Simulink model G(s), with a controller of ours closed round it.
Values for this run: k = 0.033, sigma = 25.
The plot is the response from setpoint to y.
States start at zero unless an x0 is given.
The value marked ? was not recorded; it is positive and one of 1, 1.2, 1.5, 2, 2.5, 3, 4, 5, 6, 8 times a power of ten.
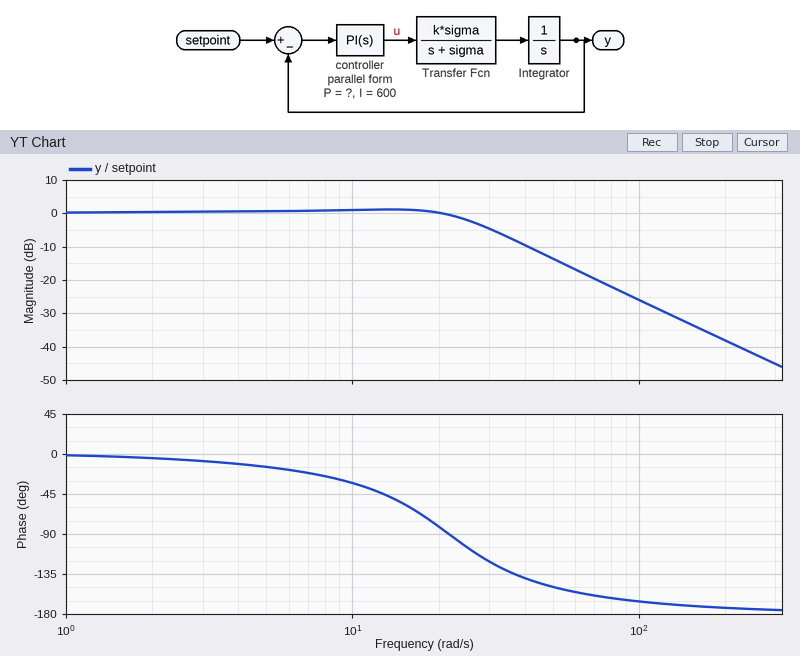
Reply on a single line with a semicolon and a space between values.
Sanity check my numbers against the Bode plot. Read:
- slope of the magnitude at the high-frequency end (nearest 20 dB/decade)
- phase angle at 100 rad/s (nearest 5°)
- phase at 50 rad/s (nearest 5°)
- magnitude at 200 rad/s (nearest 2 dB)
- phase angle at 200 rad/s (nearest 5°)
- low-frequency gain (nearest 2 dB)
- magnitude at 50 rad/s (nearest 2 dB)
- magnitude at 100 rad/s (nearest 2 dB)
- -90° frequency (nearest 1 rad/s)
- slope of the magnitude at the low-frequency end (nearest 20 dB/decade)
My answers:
-40 dB/decade; -165°; -150°; -38 dB; -175°; 0 dB; -14 dB; -26 dB; 22 rad/s; 0 dB/decade
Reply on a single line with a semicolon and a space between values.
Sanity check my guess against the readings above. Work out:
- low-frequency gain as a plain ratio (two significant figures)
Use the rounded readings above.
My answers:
1.0
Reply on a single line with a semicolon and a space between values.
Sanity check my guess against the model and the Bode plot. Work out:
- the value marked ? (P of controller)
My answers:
600
